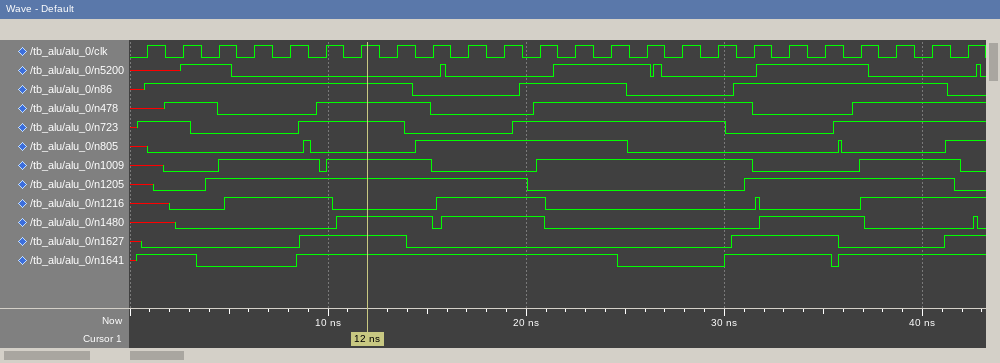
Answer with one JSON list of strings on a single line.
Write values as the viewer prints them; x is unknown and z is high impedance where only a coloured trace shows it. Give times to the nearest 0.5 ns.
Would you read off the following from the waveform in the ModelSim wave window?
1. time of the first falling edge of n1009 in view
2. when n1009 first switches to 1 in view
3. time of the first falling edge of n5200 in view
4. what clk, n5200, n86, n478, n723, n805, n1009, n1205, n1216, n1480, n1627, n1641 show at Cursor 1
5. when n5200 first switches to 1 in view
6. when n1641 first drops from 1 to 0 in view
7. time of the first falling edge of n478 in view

["9.5 ns", "4.5 ns", "5 ns", "clk=1, n5200=0, n86=1, n478=1, n723=1, n805=0, n1009=1, n1205=1, n1216=0, n1480=1, n1627=1, n1641=1", "2.5 ns", "3.5 ns", "4.5 ns"]
